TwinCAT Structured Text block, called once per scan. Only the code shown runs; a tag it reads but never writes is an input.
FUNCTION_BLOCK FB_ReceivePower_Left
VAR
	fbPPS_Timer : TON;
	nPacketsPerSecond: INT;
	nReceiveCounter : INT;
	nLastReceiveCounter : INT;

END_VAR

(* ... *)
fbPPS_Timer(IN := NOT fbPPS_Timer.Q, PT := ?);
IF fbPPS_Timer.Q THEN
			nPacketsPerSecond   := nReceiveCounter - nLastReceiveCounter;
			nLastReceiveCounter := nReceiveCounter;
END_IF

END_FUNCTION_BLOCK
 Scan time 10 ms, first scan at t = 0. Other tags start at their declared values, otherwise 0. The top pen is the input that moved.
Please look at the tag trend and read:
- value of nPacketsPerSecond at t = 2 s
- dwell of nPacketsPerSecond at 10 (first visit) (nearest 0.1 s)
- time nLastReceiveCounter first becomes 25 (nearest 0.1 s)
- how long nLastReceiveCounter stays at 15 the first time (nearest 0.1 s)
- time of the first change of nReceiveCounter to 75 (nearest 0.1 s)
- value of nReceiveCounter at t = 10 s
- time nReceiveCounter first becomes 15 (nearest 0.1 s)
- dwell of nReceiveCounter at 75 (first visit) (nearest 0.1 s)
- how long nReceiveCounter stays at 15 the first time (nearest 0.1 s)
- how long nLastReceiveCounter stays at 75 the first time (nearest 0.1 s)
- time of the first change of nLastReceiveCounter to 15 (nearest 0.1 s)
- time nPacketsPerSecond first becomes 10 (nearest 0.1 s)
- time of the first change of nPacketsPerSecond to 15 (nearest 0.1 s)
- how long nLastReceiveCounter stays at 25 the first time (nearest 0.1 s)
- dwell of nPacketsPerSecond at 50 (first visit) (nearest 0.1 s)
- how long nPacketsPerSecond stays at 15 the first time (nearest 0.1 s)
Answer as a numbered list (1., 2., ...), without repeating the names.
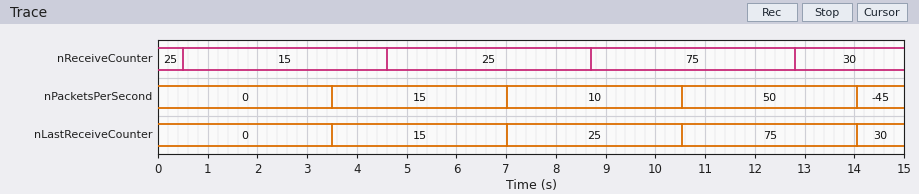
1. 0
2. 3.5 s
3. 7.0 s
4. 3.5 s
5. 8.7 s
6. 75
7. 0.5 s
8. 4.1 s
9. 4.1 s
10. 3.5 s
11. 3.5 s
12. 7.0 s
13. 3.5 s
14. 3.5 s
15. 3.5 s
16. 3.5 s
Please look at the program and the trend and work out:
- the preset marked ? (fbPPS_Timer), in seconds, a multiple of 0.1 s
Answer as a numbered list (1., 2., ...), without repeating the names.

1. 3.5 s
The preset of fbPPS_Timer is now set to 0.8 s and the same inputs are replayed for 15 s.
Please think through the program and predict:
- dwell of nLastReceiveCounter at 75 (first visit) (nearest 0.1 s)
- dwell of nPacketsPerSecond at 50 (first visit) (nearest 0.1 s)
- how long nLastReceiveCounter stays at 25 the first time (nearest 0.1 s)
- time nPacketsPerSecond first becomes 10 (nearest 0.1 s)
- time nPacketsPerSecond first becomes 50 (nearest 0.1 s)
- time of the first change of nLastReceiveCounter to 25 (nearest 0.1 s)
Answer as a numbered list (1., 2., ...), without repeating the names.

1. 4.1 s
2. 0.8 s
3. 4.1 s
4. 4.9 s
5. 9.0 s
6. 4.9 s
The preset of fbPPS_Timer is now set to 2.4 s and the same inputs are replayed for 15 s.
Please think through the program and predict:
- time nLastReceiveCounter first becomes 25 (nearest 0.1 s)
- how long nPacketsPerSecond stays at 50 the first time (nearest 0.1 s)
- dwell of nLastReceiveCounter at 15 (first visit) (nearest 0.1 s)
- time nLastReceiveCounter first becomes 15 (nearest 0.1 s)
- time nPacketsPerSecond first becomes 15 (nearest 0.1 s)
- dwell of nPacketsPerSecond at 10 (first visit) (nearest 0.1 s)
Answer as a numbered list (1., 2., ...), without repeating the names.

1. 4.8 s
2. 2.4 s
3. 2.4 s
4. 2.4 s
5. 2.4 s
6. 2.4 s
